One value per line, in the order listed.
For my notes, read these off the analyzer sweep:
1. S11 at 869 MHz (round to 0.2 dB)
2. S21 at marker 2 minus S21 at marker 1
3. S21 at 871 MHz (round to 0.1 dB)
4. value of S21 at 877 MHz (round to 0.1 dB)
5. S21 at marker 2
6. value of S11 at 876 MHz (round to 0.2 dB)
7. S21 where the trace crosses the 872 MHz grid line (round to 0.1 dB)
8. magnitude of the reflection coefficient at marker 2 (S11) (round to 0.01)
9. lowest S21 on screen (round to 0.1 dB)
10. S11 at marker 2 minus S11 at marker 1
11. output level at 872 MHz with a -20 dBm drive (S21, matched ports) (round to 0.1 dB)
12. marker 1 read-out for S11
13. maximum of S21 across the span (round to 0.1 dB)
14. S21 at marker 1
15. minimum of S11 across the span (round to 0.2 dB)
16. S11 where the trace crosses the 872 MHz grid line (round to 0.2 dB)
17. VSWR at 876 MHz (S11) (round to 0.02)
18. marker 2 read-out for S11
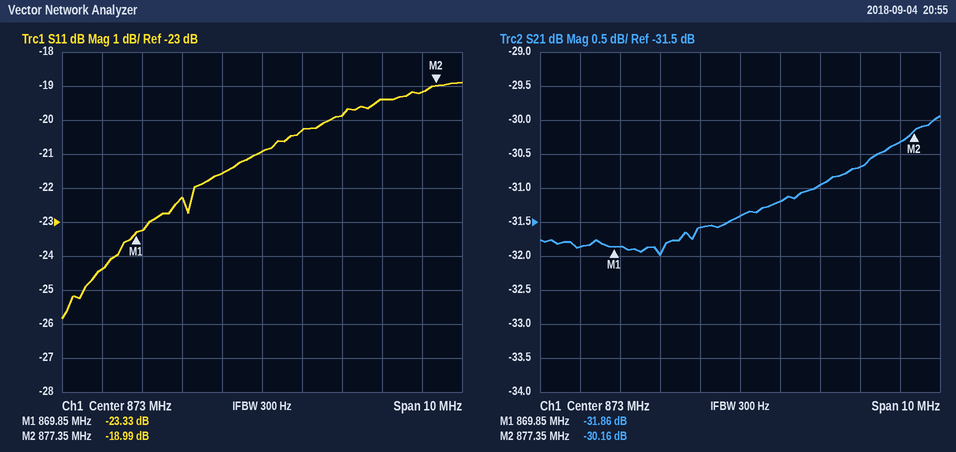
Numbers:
-24.4 dB
1.70 dB
-32.0 dB
-30.3 dB
-30.16 dB
-19.4 dB
-31.6 dB
0.11
-32.0 dB
4.34 dB
-51.6 dBm
-23.33 dB
-29.9 dB
-31.86 dB
-25.8 dB
-21.6 dB
1.24
-18.99 dB
